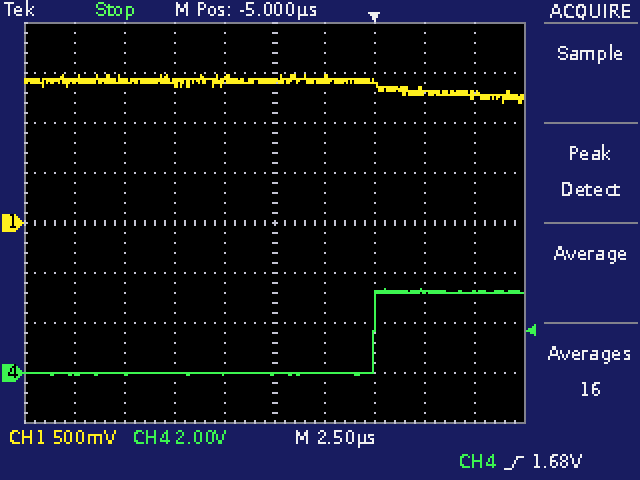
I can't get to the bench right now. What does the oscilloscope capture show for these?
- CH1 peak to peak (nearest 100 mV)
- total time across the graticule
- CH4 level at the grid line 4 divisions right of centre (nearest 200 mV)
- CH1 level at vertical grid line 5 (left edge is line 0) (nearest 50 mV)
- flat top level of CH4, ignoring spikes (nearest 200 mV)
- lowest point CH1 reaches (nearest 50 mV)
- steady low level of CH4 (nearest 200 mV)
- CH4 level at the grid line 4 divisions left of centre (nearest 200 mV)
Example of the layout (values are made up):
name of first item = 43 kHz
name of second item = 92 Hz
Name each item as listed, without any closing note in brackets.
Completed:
CH1 peak to peak = 300 mV
total time across the graticule = 25 µs
CH4 level at the grid line 4 divisions right of centre = 3.2 V
CH1 level at vertical grid line 5 (left edge is line 0) = 1.40 V
flat top level of CH4, ignoring spikes = 3.2 V
lowest point CH1 reaches = 1.20 V
steady low level of CH4 = 0.0 V
CH4 level at the grid line 4 divisions left of centre = 0.0 V
